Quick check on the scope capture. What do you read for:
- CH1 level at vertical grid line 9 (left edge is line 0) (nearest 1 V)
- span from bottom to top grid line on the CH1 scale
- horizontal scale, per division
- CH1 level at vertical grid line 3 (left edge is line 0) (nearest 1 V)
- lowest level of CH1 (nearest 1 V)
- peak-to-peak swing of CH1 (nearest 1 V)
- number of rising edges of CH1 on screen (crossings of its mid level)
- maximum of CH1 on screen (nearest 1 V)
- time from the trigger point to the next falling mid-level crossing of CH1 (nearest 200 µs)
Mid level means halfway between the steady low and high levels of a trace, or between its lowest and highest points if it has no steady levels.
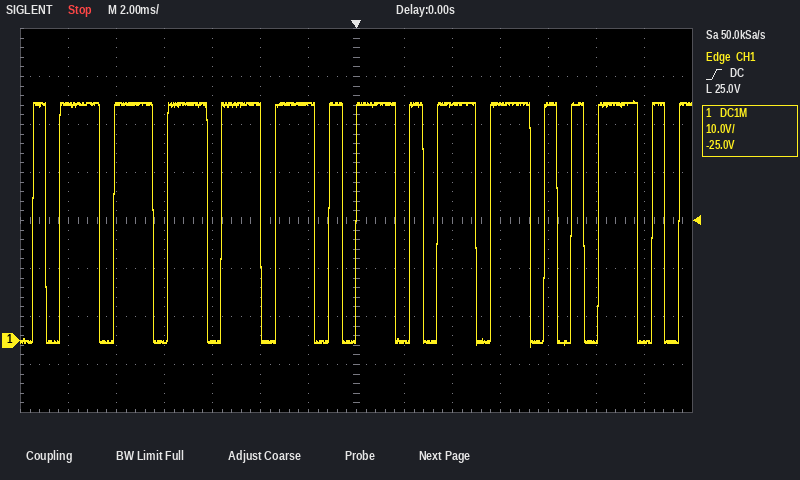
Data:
49 V
80 V
2 ms
0 V
-1 V
51 V
16
50 V
1.6 ms
